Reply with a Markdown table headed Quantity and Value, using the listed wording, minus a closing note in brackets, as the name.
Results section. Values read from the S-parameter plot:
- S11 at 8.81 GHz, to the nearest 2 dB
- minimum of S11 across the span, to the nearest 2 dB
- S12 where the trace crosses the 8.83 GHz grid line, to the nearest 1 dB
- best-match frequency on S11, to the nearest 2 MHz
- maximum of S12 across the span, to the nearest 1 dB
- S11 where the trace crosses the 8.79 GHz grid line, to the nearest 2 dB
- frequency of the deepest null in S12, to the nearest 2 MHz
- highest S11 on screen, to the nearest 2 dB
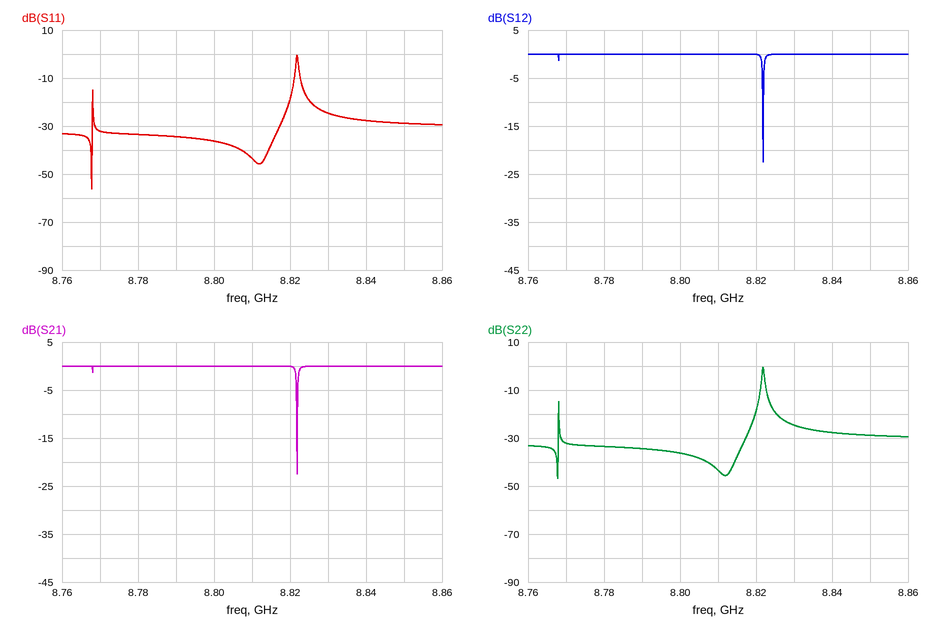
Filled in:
| Quantity | Value |
|---|---|
| S11 at 8.81 GHz, to the nearest 2 dB | -44 dB |
| minimum of S11 across the span, to the nearest 2 dB | -56 dB |
| S12 where the trace crosses the 8.83 GHz grid line, to the nearest 1 dB | 0 dB |
| best-match frequency on S11, to the nearest 2 MHz | 8.768 GHz |
| maximum of S12 across the span, to the nearest 1 dB | 0 dB |
| S11 where the trace crosses the 8.79 GHz grid line, to the nearest 2 dB | -34 dB |
| frequency of the deepest null in S12, to the nearest 2 MHz | 8.822 GHz |
| highest S11 on screen, to the nearest 2 dB | 0 dB |
